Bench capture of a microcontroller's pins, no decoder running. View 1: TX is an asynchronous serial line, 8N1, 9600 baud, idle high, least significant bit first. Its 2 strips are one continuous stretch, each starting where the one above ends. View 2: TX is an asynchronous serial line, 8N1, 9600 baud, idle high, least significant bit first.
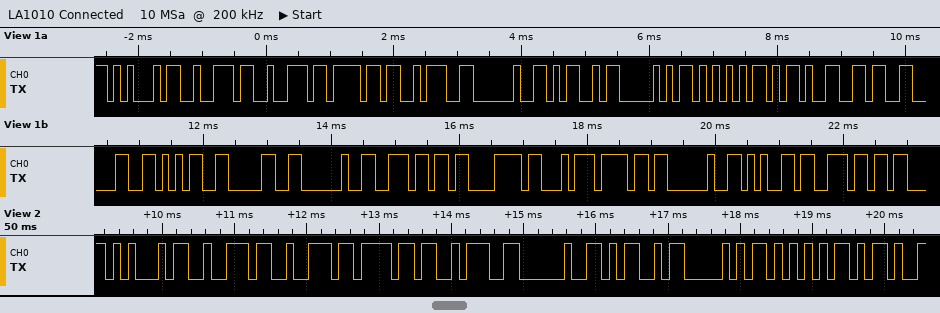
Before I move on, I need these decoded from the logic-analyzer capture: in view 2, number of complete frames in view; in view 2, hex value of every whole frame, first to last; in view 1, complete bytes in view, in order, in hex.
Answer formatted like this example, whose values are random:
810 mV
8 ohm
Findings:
10
45 72 72 6F 3A 20 4D 50 55 2D
45 72 72 6F 3A 20 4D 50 55 2D 36 30 35 30 20 6E C3 A3 6F 20 65 6E
